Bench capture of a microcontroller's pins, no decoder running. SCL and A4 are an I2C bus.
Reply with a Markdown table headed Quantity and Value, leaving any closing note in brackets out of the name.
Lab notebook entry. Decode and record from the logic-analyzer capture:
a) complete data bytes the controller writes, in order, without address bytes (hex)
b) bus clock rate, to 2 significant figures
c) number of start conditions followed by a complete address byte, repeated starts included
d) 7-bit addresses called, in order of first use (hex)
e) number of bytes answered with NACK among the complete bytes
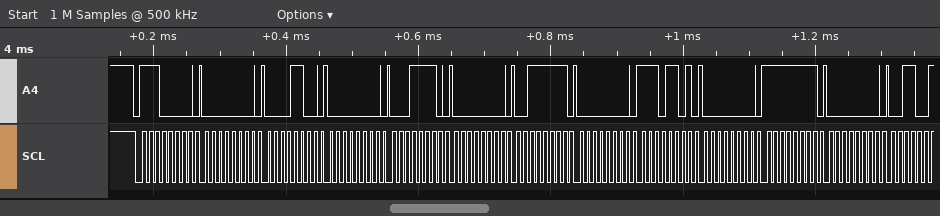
| Quantity | Value |
|---|---|
| complete data bytes the controller writes, in order, without address bytes | 00 0C 00 1E 00 3F 00 ED 00 FF 00 |
| bus clock rate, to 2 significant figures | 100 kHz |
| number of start conditions followed by a complete address byte, repeated starts included | 1 |
| 7-bit addresses called, in order of first use | 0x70 |
| number of bytes answered with NACK among the complete bytes | 0 |
